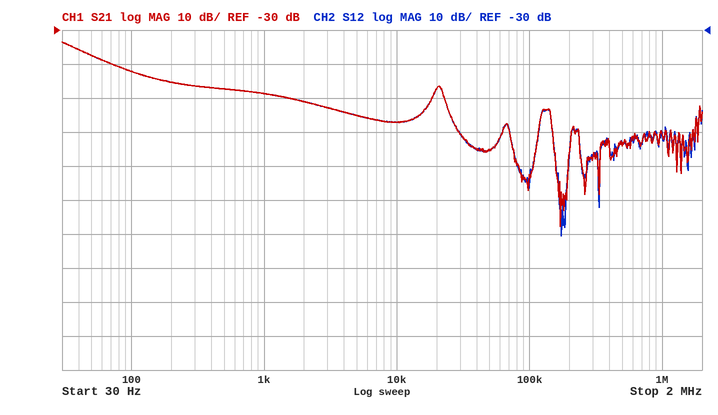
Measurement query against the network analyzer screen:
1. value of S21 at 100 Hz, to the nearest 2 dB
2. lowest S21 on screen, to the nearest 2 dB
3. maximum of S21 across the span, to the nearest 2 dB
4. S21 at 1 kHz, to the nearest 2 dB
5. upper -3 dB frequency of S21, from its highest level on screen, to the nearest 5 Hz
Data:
-42 dB
-88 dB
-34 dB
-48 dB
45 Hz
